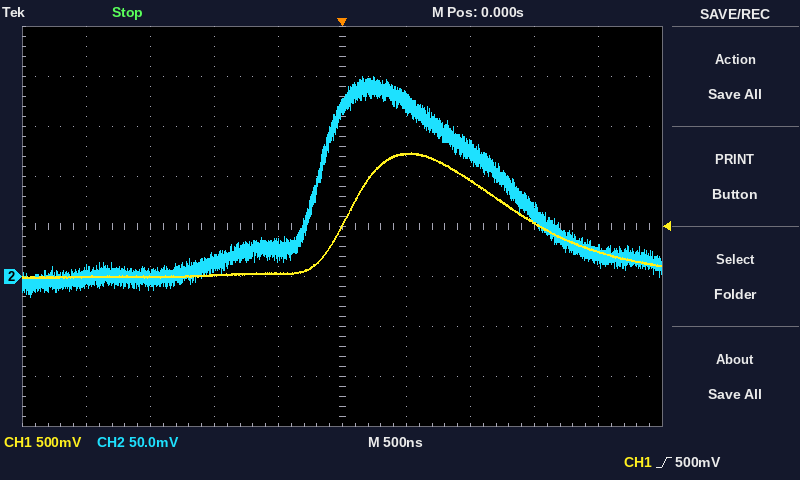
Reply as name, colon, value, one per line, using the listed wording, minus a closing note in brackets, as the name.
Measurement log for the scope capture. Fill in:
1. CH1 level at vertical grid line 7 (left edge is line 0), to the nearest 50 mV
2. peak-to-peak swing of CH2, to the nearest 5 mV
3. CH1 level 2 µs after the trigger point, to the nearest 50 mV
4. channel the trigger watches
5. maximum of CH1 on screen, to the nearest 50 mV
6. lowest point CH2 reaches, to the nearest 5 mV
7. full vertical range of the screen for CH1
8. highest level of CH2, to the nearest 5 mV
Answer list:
CH1 level at vertical grid line 7 (left edge is line 0), to the nearest 50 mV: 950 mV
peak-to-peak swing of CH2, to the nearest 5 mV: 220 mV
CH1 level 2 µs after the trigger point, to the nearest 50 mV: 250 mV
channel the trigger watches: CH1
maximum of CH1 on screen, to the nearest 50 mV: 1.25 V
lowest point CH2 reaches, to the nearest 5 mV: -20 mV
full vertical range of the screen for CH1: 4 V
highest level of CH2, to the nearest 5 mV: 200 mV
